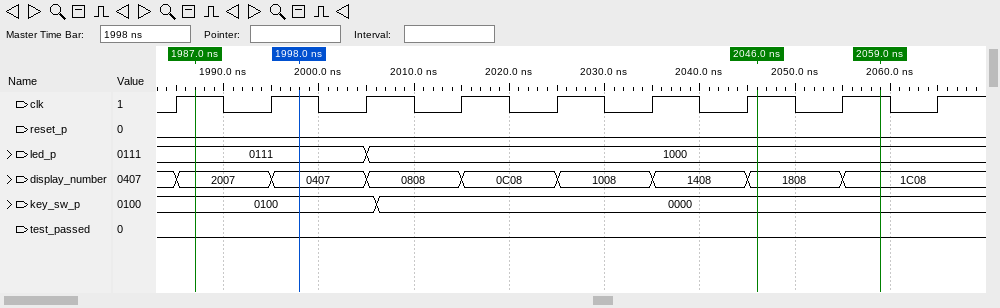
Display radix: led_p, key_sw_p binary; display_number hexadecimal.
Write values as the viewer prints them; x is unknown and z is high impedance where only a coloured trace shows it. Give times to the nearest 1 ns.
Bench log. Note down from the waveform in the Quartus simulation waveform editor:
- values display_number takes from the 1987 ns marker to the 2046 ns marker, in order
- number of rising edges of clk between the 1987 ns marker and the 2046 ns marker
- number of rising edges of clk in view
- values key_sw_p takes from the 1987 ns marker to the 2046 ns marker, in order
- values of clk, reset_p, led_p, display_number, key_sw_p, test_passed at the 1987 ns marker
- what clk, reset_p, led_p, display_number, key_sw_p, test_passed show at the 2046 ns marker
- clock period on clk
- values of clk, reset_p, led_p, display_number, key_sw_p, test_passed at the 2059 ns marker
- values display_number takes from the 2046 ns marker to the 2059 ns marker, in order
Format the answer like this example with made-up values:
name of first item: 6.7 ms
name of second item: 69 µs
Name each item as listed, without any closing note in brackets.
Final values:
values display_number takes from the 1987 ns marker to the 2046 ns marker, in order: 2007, 0407, 0808, 0C08, 1008, 1408, 1808
number of rising edges of clk between the 1987 ns marker and the 2046 ns marker: 6
number of rising edges of clk in view: 9
values key_sw_p takes from the 1987 ns marker to the 2046 ns marker, in order: 0100, 0000
values of clk, reset_p, led_p, display_number, key_sw_p, test_passed at the 1987 ns marker: clk=1, reset_p=0, led_p=0111, display_number=2007, key_sw_p=0100, test_passed=0
what clk, reset_p, led_p, display_number, key_sw_p, test_passed show at the 2046 ns marker: clk=1, reset_p=0, led_p=1000, display_number=1808, key_sw_p=0000, test_passed=0
clock period on clk: 10 ns
values of clk, reset_p, led_p, display_number, key_sw_p, test_passed at the 2059 ns marker: clk=1, reset_p=0, led_p=1000, display_number=1C08, key_sw_p=0000, test_passed=0
values display_number takes from the 2046 ns marker to the 2059 ns marker, in order: 1808, 1C08
